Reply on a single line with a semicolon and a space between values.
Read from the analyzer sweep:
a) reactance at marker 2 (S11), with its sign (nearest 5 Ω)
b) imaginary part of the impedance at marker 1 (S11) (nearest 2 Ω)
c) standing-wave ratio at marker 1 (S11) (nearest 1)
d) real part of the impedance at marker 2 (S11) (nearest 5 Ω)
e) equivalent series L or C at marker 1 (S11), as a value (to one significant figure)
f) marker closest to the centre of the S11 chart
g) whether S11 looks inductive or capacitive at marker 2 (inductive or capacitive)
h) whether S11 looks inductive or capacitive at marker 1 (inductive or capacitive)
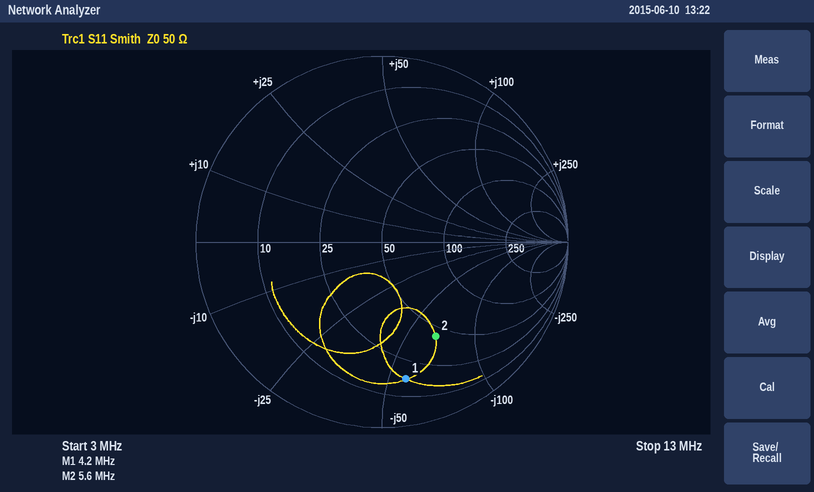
-65 Ω; -56 Ω; 7; 45 Ω; 700 pF; marker 2; capacitive; capacitive
